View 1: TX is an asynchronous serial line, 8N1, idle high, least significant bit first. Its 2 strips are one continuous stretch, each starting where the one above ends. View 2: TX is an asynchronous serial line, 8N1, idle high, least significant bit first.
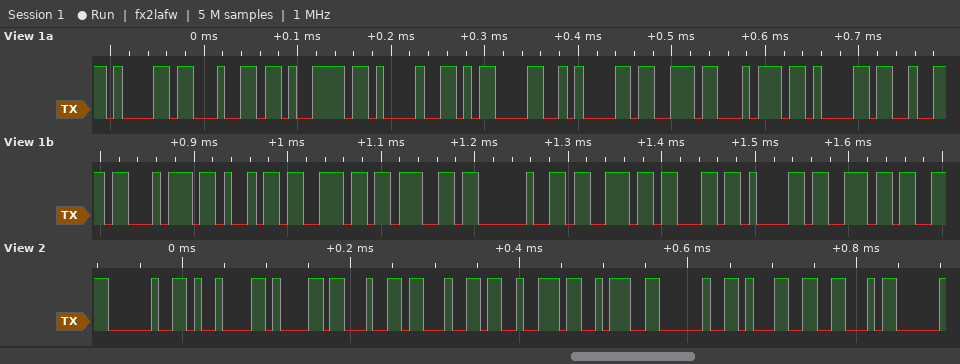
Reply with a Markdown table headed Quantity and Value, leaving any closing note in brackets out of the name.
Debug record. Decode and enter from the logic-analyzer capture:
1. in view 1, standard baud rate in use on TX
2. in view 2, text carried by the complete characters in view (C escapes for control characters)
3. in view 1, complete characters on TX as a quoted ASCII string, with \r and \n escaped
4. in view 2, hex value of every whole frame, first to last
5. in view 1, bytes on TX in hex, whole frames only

| Quantity | Value |
|---|---|
| in view 1, standard baud rate in use on TX | 115200 baud |
| in view 2, text carried by the complete characters in view | " \taddr: 1F" |
| in view 1, complete characters on TX as a quoted ASCII string, with \r and \n escaped | "ady!\r\nstarting scan" |
| in view 2, hex value of every whole frame, first to last | 20 09 61 64 64 72 3A 20 31 46 |
| in view 1, bytes on TX in hex, whole frames only | 61 64 79 21 0D 0A 73 74 61 72 74 69 6E 67 20 73 63 61 6E |
